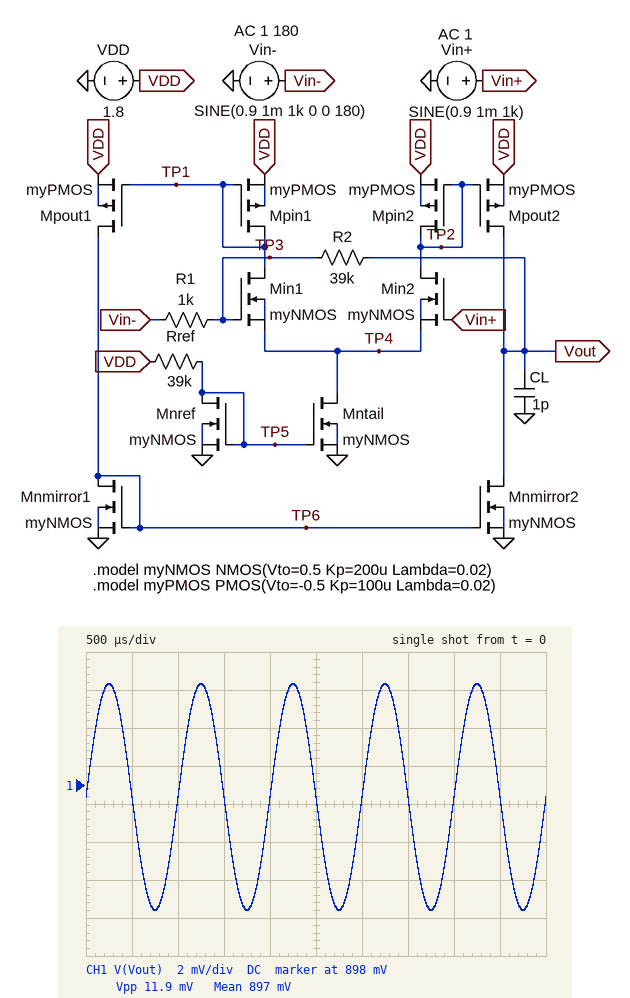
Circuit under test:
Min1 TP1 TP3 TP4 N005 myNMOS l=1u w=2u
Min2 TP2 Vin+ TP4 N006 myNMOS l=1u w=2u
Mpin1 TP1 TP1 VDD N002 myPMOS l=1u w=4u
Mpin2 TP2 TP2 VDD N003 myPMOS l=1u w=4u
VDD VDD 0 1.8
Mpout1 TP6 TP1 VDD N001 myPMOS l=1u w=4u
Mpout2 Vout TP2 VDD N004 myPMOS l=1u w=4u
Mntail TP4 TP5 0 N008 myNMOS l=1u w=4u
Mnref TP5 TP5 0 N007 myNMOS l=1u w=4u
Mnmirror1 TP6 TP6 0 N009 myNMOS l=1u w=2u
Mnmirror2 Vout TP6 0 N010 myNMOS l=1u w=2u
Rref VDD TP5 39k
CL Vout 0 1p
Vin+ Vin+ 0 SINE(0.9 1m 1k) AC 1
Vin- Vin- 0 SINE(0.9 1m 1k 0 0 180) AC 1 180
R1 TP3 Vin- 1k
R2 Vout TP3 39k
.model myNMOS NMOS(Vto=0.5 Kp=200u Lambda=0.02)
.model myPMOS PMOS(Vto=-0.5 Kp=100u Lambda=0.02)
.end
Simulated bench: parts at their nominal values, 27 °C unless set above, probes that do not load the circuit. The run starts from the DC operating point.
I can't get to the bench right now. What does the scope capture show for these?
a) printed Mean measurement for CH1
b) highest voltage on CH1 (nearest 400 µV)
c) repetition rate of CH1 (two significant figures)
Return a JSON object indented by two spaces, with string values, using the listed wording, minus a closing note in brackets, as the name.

{
  "printed Mean measurement for CH1": "897 mV",
  "highest voltage on CH1": "903.2 mV",
  "repetition rate of CH1": "1.0 kHz"
}
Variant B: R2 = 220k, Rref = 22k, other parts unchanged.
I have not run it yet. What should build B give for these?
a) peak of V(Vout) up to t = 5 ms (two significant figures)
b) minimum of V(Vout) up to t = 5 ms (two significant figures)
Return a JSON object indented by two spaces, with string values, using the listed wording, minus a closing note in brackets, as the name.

{
  "peak of V(Vout) up to t = 5 ms": "920 mV",
  "minimum of V(Vout) up to t = 5 ms": "850 mV"
}
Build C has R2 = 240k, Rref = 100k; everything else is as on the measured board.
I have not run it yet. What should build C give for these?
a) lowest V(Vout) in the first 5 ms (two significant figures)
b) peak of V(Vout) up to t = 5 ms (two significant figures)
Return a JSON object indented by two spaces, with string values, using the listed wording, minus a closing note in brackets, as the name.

{
  "lowest V(Vout) in the first 5 ms": "860 mV",
  "peak of V(Vout) up to t = 5 ms": "920 mV"
}
